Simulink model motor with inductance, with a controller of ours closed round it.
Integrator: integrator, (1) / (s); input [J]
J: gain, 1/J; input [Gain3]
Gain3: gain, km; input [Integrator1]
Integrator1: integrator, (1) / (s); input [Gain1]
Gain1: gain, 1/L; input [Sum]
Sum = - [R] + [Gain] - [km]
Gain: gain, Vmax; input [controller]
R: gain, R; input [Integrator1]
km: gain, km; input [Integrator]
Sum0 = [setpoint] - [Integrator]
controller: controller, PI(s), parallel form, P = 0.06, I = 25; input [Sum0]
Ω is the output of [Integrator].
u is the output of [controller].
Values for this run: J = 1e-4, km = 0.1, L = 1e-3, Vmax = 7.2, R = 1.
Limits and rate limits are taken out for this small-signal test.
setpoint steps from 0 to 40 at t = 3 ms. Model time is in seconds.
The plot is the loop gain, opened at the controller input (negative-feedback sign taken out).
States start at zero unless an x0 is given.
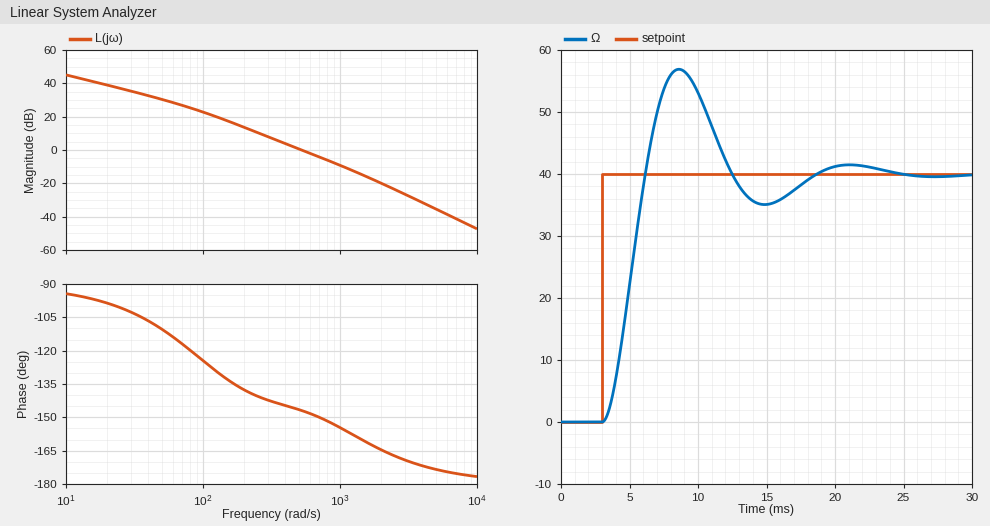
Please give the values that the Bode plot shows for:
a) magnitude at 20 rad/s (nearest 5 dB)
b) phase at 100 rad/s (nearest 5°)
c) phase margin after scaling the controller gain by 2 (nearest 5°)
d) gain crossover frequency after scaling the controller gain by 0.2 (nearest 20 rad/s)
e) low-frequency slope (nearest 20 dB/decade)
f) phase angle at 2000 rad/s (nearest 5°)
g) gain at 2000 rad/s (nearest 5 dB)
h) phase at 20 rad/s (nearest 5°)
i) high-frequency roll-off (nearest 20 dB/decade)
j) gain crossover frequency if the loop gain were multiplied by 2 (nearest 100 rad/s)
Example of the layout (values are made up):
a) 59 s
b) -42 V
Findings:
a) 40 dB
b) -125°
c) 30°
d) 200 rad/s
e) -20 dB/decade
f) -165°
g) -20 dB
h) -100°
i) -40 dB/decade
j) 800 rad/s
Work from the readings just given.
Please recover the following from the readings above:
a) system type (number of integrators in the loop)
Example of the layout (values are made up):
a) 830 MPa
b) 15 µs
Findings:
a) 1
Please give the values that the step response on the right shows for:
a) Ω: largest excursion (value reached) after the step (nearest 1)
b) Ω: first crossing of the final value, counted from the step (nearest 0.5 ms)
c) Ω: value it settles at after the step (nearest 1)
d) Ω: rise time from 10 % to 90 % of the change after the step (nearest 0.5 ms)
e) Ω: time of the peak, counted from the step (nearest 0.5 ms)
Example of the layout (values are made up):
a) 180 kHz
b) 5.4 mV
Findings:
a) 57
b) 3.0 ms
c) 40
d) 2.0 ms
e) 5.5 ms
